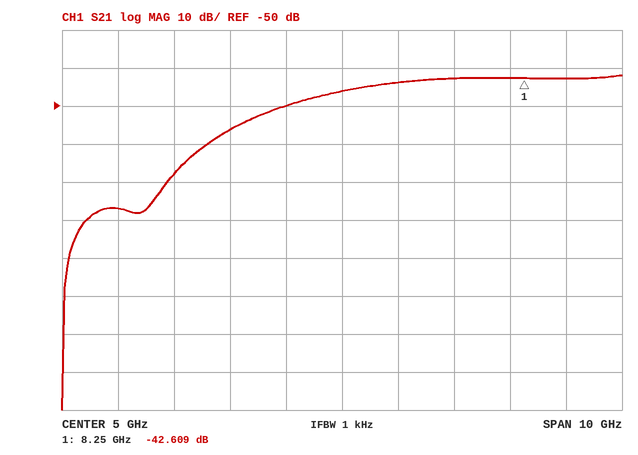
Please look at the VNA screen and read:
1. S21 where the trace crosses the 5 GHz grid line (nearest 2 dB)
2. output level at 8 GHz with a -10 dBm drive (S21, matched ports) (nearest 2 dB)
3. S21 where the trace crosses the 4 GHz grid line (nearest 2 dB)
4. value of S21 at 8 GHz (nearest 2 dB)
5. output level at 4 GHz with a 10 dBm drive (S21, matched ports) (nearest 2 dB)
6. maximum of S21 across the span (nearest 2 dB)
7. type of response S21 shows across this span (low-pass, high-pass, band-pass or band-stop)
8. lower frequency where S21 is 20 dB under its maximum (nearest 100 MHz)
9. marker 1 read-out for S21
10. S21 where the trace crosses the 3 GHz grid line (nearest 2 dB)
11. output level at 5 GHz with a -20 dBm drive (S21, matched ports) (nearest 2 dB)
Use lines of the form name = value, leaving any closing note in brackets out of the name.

S21 where the trace crosses the 5 GHz grid line = -46 dB
output level at 8 GHz with a -10 dBm drive (S21, matched ports) = -52 dBm
S21 where the trace crosses the 4 GHz grid line = -50 dB
value of S21 at 8 GHz = -42 dB
output level at 4 GHz with a 10 dBm drive (S21, matched ports) = -40 dBm
maximum of S21 across the span = -42 dB
type of response S21 shows across this span = high-pass
lower frequency where S21 is 20 dB under its maximum = 2.4 GHz
marker 1 read-out for S21 = -42.609 dB
S21 where the trace crosses the 3 GHz grid line = -56 dB
output level at 5 GHz with a -20 dBm drive (S21, matched ports) = -66 dBm
